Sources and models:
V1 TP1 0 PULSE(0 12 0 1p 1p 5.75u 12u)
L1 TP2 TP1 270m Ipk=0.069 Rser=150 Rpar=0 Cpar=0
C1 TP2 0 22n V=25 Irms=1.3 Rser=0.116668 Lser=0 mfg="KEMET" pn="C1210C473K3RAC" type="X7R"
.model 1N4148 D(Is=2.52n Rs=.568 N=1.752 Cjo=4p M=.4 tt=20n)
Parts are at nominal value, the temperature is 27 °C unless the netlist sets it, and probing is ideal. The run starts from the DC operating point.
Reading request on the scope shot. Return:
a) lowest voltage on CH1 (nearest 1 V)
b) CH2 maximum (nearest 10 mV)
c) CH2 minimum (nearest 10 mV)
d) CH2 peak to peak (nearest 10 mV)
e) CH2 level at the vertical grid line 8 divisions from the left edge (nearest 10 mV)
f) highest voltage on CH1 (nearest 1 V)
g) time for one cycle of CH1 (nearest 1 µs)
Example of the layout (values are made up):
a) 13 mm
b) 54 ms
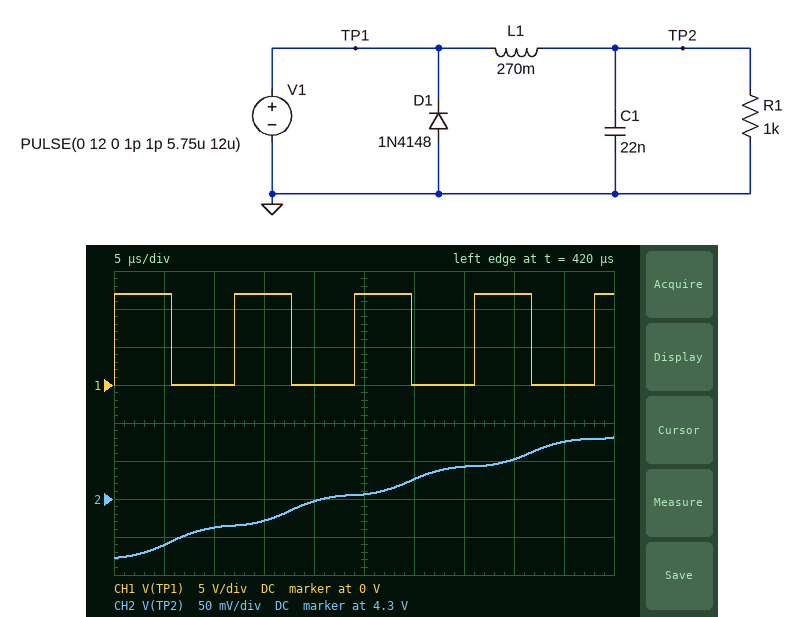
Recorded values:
a) 0 V
b) 4.38 V
c) 4.22 V
d) 160 mV
e) 4.35 V
f) 12 V
g) 12 µs
